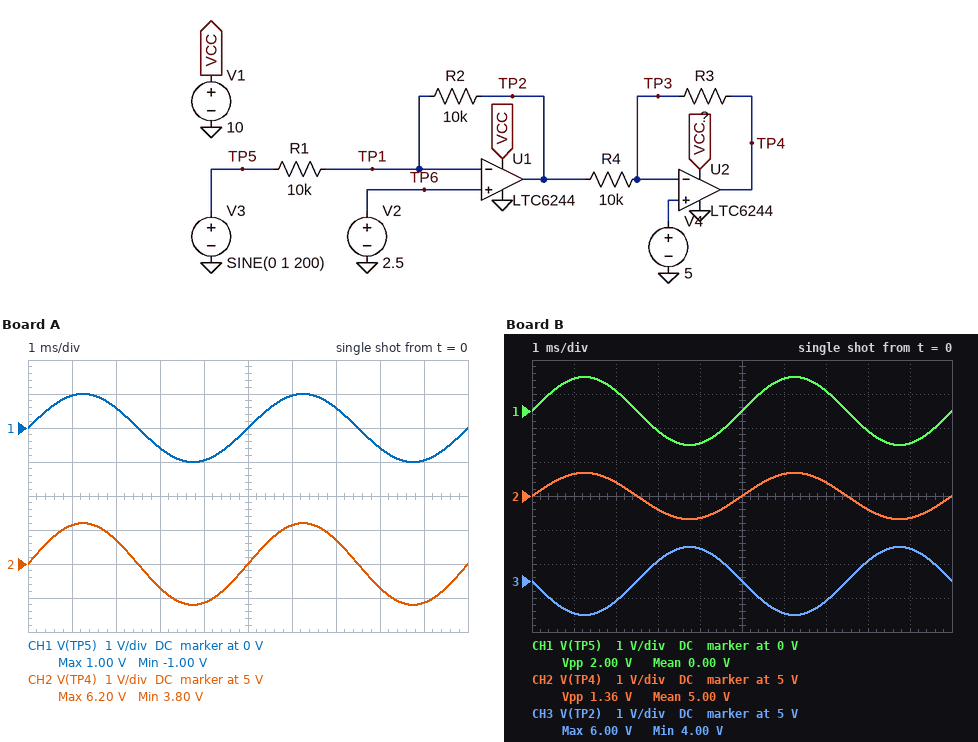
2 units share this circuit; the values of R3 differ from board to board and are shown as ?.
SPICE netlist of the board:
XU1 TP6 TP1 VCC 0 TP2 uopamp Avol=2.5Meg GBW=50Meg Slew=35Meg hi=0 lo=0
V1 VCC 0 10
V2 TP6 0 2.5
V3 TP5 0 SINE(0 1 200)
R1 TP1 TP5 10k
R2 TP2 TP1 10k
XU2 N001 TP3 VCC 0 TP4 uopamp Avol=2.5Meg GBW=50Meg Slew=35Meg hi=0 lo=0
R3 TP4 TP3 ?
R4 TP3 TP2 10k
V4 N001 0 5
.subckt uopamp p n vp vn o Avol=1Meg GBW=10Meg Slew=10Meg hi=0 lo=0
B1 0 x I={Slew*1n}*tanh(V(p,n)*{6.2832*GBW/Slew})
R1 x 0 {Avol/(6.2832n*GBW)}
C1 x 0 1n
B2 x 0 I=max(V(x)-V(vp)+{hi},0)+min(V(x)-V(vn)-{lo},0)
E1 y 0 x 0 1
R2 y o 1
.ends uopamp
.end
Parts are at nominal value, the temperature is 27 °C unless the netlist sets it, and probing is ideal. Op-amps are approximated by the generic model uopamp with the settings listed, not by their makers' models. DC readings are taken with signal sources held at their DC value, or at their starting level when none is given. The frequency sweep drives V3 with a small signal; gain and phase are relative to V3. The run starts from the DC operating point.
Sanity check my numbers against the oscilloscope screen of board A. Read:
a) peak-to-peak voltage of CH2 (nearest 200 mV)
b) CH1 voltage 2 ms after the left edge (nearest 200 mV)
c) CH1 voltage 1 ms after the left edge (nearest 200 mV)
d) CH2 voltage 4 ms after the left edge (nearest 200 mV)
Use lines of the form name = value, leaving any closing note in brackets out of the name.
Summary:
peak-to-peak voltage of CH2 = 2.4 V
CH1 voltage 2 ms after the left edge = 600 mV
CH1 voltage 1 ms after the left edge = 1.0 V
CH2 voltage 4 ms after the left edge = 3.8 V
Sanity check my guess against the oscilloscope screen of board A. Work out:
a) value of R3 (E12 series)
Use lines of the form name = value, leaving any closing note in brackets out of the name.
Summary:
value of R3 = 12 kΩ
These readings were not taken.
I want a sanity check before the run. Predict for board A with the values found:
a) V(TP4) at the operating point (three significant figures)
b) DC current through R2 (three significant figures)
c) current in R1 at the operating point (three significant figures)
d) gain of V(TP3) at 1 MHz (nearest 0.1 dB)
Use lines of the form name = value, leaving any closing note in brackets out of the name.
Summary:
V(TP4) at the operating point = 5.00 V
DC current through R2 = 250 µA
current in R1 at the operating point = 250 µA
gain of V(TP3) at 1 MHz = -32.4 dB
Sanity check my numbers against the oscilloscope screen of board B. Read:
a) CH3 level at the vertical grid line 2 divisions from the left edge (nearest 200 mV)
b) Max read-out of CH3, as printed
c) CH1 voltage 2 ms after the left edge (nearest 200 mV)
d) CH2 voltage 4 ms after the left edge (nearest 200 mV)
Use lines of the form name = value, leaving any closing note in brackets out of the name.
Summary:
CH3 level at the vertical grid line 2 divisions from the left edge = 4.4 V
Max read-out of CH3, as printed = 6.00 V
CH1 voltage 2 ms after the left edge = 600 mV
CH2 voltage 4 ms after the left edge = 4.4 V
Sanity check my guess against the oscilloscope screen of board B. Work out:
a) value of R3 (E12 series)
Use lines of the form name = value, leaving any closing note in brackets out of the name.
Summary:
value of R3 = 6.8 kΩ
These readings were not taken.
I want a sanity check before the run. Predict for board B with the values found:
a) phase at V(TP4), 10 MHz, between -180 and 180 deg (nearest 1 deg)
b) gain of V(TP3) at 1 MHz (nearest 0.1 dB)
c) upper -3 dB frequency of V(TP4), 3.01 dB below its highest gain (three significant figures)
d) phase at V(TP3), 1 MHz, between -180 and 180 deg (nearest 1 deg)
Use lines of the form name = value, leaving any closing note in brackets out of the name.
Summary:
phase at V(TP4), 10 MHz, between -180 and 180 deg = -40 deg
gain of V(TP3) at 1 MHz = -37.3 dB
upper -3 dB frequency of V(TP4), 3.01 dB below its highest gain = 17.5 MHz
phase at V(TP3), 1 MHz, between -180 and 180 deg = -94 deg
